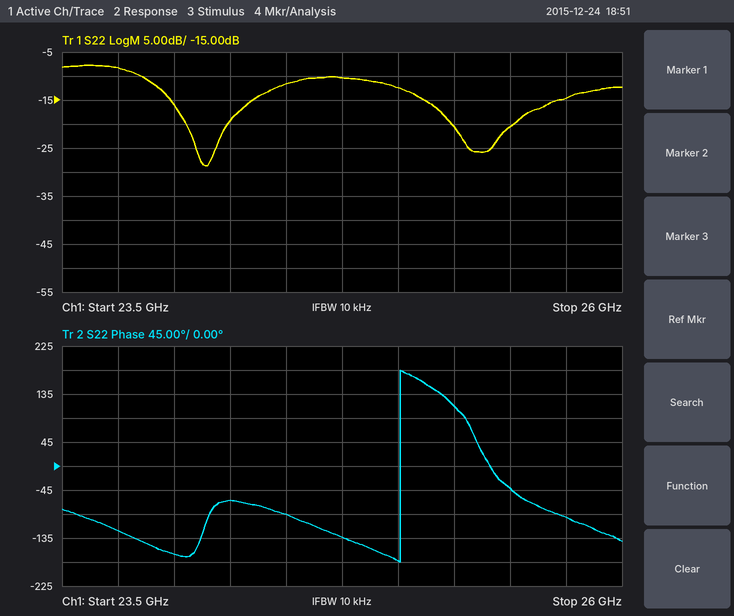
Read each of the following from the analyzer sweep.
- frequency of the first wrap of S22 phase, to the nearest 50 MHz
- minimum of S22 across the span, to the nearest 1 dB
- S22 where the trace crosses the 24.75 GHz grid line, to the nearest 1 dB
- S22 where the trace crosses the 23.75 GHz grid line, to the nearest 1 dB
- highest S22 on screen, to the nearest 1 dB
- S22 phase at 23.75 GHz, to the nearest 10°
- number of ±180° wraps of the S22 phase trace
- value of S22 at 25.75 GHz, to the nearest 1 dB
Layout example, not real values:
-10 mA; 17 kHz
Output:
25.00 GHz; -29 dB; -10 dB; -8 dB; -8 dB; -120°; 1; -15 dB
